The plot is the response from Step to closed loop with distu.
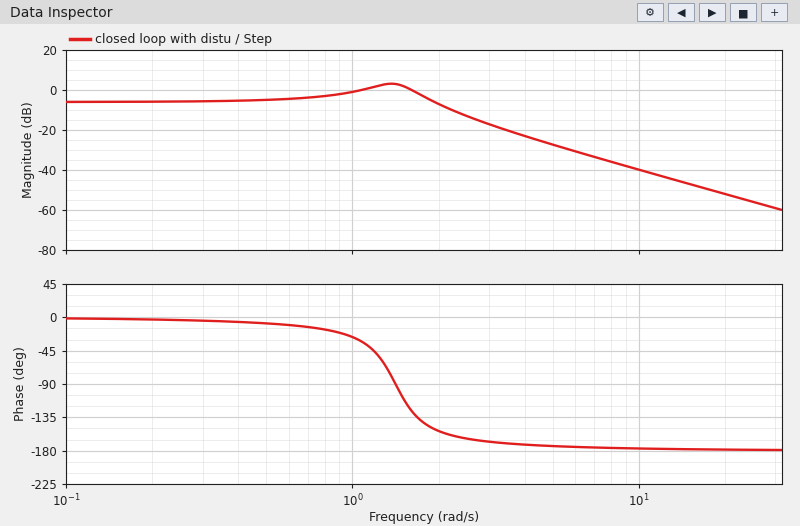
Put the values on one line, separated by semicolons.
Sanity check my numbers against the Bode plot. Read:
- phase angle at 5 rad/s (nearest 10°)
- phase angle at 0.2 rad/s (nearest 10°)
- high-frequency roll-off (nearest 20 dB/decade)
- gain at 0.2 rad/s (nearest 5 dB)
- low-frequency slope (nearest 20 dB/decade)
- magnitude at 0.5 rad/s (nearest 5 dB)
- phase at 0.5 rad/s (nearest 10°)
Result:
-170°; 0°; -40 dB/decade; -5 dB; 0 dB/decade; -5 dB; -10°
